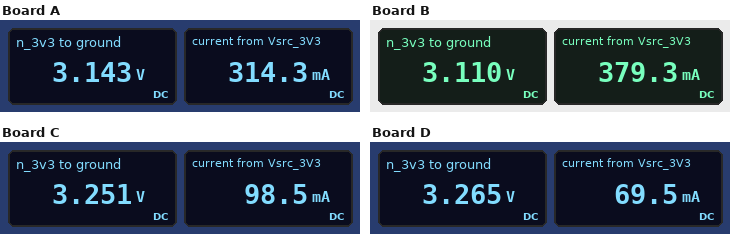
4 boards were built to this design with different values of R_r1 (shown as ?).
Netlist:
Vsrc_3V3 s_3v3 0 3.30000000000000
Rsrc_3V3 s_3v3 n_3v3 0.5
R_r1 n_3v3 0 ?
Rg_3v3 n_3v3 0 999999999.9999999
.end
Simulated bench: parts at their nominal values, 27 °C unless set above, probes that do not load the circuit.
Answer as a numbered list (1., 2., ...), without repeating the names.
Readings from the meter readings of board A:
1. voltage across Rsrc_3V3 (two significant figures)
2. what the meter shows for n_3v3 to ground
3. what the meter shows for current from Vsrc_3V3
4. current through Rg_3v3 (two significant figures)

1. 160 mV
2. 3.143 V
3. 314.3 mA
4. 3.1 nA
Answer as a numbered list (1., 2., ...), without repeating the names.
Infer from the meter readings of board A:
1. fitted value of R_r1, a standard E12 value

1. 10 Ω
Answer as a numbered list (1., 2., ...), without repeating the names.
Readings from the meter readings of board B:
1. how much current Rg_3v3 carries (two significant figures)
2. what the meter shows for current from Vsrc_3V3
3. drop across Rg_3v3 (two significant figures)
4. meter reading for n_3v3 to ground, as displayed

1. 3.1 nA
2. 379.3 mA
3. 3.1 V
4. 3.110 V
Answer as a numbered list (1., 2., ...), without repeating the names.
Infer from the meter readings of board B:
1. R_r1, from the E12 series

1. 8.2 Ω
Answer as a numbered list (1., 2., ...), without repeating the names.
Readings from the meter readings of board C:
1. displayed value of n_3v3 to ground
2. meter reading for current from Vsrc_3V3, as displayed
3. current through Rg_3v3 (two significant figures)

1. 3.251 V
2. 98.5 mA
3. 3.3 nA
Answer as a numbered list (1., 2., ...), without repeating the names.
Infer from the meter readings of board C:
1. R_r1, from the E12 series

1. 33 Ω
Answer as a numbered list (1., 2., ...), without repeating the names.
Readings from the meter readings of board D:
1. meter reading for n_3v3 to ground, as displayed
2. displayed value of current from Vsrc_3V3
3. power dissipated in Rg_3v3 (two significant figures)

1. 3.265 V
2. 69.5 mA
3. 11 nW
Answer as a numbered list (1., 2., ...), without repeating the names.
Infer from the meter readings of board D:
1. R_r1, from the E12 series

1. 47 Ω
